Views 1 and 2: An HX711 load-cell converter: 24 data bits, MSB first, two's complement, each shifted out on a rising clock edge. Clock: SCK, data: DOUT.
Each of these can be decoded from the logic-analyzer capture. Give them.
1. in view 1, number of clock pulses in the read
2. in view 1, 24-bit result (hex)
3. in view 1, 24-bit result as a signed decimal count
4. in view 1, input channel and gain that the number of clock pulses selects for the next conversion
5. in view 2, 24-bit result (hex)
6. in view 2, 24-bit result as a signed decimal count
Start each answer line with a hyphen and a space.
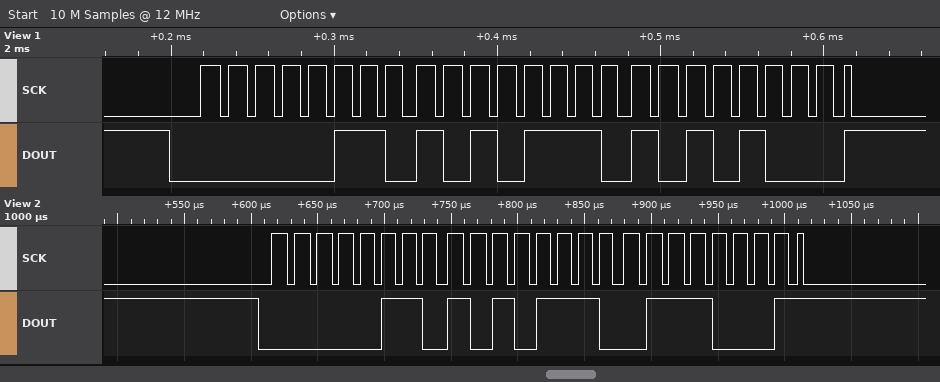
- 25
- 0x06AEA8
- 437928
- channel A, gain 128
- 0x06AE71
- 437873
